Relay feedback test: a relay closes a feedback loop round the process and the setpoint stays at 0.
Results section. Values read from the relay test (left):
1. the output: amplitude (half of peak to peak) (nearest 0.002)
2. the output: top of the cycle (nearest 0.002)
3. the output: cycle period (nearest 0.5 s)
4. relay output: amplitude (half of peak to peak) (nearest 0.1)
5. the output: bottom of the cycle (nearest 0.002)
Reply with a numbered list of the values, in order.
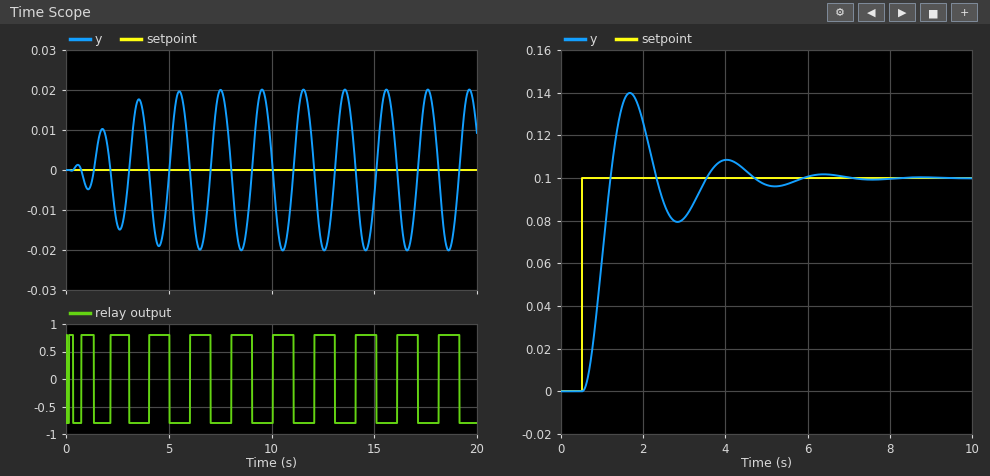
1. 0.020
2. 0.020
3. 2.0 s
4. 0.8
5. -0.020
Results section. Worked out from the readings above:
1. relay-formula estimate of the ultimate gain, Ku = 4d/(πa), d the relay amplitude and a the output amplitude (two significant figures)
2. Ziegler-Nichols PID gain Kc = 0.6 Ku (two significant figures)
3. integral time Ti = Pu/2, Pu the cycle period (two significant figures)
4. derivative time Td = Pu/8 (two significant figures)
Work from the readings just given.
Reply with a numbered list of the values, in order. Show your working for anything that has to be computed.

1. 4 × 0.8 / (π × 0.02) = 51
2. 0.6 × 51 = 31
3. 2 / 2 = 1.0 s
4. 2 / 8 = 0.25 s
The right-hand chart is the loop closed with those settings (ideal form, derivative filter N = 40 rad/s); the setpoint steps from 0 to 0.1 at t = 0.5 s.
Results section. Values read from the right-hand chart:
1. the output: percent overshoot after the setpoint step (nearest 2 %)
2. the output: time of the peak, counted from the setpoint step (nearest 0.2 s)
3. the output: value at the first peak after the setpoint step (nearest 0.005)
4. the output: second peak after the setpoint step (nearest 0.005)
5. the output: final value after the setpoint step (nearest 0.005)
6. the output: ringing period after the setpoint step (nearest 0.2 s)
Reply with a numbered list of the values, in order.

1. 40 %
2. 1.2 s
3. 0.140
4. 0.110
5. 0.100
6. 2.4 s
